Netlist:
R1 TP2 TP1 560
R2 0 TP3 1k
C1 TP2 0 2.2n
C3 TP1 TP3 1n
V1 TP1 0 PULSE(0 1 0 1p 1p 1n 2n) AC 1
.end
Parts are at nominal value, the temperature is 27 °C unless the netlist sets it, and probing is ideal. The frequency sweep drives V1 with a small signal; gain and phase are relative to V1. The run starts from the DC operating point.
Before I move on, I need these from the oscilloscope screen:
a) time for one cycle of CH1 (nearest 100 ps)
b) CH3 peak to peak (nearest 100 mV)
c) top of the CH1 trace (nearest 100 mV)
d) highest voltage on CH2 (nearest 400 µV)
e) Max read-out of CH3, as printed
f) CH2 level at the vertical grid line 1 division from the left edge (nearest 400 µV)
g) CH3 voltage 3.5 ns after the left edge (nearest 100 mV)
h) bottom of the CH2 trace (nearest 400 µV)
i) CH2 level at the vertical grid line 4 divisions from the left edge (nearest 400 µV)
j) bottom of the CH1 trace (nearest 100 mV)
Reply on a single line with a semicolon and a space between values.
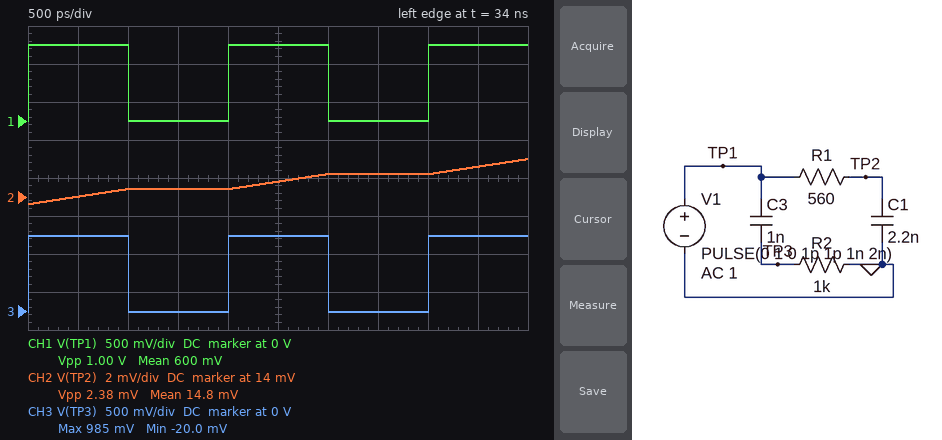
2.0 ns; 1.0 V; 1.0 V; 16.0 mV; 985 mV; 14.0 mV; 0 V; 13.6 mV; 14.4 mV; 0 V
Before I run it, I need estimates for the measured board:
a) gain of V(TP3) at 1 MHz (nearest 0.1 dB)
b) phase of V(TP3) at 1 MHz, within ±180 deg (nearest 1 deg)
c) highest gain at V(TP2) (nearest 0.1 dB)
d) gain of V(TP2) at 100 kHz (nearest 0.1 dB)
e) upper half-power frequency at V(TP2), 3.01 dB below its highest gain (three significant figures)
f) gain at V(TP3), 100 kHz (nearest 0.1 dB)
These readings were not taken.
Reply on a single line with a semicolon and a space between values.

-0.1 dB; 9 deg; 0 dB; -2.0 dB; 129 kHz; -5.5 dB
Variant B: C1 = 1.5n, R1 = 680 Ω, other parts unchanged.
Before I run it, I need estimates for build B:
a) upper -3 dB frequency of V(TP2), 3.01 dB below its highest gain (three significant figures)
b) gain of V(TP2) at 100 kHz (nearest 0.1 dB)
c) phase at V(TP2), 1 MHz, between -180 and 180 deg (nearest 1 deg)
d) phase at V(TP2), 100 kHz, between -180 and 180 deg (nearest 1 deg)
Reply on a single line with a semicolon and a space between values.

156 kHz; -1.5 dB; -81 deg; -33 deg
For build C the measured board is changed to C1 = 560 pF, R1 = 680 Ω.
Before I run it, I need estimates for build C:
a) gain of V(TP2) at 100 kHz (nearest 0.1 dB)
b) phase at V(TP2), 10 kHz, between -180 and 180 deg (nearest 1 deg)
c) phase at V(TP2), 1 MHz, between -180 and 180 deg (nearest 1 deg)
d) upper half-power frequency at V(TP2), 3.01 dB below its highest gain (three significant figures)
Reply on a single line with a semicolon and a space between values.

-0.2 dB; -1 deg; -67 deg; 418 kHz
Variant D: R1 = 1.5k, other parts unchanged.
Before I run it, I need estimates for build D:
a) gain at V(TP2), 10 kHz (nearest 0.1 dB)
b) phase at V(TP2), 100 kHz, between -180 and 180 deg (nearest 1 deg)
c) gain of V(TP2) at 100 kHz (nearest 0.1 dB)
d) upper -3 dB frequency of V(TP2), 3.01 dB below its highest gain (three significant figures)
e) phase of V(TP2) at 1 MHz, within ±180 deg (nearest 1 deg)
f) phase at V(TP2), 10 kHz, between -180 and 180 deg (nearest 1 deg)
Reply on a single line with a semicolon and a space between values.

-0.2 dB; -64 deg; -7.2 dB; 48.2 kHz; -87 deg; -12 deg
